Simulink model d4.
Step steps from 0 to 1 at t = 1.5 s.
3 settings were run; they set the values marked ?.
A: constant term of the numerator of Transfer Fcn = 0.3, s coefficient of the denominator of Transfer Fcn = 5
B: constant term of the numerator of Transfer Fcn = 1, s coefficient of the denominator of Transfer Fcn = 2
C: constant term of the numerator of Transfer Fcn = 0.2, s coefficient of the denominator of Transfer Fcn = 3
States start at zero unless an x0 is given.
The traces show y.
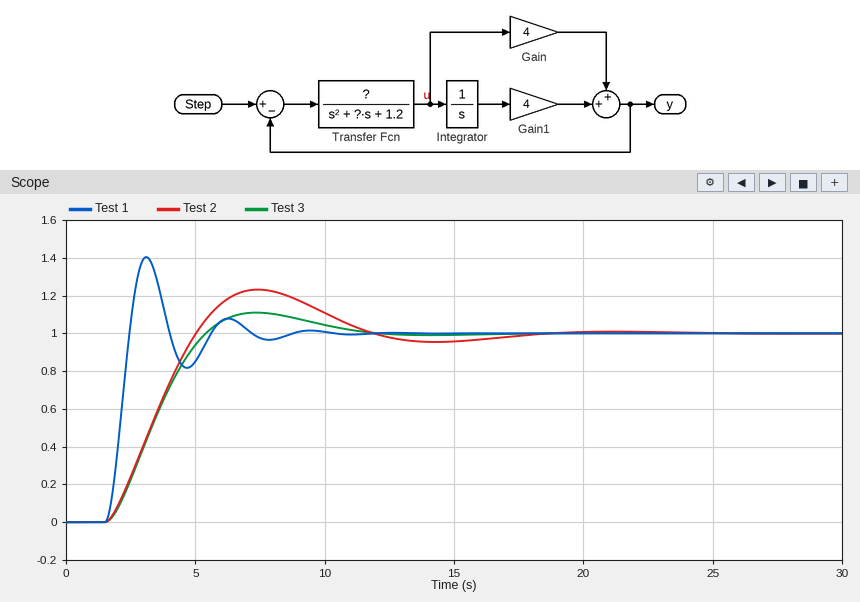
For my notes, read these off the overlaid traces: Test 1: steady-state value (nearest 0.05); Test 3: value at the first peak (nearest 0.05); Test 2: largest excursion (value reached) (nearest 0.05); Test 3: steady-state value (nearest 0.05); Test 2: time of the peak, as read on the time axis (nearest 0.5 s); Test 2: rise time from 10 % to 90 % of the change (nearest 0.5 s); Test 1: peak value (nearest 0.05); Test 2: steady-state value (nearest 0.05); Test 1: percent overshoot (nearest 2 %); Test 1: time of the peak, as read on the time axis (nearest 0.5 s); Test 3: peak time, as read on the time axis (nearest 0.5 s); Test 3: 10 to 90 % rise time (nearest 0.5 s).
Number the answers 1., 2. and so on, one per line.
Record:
1. 1.00
2. 1.10
3. 1.25
4. 1.00
5. 7.5 s
6. 2.5 s
7. 1.40
8. 1.00
9. 40 %
10. 3.0 s
11. 7.5 s
12. 2.5 s
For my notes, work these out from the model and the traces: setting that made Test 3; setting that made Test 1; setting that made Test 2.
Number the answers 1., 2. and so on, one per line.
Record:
1. C
2. B
3. A
